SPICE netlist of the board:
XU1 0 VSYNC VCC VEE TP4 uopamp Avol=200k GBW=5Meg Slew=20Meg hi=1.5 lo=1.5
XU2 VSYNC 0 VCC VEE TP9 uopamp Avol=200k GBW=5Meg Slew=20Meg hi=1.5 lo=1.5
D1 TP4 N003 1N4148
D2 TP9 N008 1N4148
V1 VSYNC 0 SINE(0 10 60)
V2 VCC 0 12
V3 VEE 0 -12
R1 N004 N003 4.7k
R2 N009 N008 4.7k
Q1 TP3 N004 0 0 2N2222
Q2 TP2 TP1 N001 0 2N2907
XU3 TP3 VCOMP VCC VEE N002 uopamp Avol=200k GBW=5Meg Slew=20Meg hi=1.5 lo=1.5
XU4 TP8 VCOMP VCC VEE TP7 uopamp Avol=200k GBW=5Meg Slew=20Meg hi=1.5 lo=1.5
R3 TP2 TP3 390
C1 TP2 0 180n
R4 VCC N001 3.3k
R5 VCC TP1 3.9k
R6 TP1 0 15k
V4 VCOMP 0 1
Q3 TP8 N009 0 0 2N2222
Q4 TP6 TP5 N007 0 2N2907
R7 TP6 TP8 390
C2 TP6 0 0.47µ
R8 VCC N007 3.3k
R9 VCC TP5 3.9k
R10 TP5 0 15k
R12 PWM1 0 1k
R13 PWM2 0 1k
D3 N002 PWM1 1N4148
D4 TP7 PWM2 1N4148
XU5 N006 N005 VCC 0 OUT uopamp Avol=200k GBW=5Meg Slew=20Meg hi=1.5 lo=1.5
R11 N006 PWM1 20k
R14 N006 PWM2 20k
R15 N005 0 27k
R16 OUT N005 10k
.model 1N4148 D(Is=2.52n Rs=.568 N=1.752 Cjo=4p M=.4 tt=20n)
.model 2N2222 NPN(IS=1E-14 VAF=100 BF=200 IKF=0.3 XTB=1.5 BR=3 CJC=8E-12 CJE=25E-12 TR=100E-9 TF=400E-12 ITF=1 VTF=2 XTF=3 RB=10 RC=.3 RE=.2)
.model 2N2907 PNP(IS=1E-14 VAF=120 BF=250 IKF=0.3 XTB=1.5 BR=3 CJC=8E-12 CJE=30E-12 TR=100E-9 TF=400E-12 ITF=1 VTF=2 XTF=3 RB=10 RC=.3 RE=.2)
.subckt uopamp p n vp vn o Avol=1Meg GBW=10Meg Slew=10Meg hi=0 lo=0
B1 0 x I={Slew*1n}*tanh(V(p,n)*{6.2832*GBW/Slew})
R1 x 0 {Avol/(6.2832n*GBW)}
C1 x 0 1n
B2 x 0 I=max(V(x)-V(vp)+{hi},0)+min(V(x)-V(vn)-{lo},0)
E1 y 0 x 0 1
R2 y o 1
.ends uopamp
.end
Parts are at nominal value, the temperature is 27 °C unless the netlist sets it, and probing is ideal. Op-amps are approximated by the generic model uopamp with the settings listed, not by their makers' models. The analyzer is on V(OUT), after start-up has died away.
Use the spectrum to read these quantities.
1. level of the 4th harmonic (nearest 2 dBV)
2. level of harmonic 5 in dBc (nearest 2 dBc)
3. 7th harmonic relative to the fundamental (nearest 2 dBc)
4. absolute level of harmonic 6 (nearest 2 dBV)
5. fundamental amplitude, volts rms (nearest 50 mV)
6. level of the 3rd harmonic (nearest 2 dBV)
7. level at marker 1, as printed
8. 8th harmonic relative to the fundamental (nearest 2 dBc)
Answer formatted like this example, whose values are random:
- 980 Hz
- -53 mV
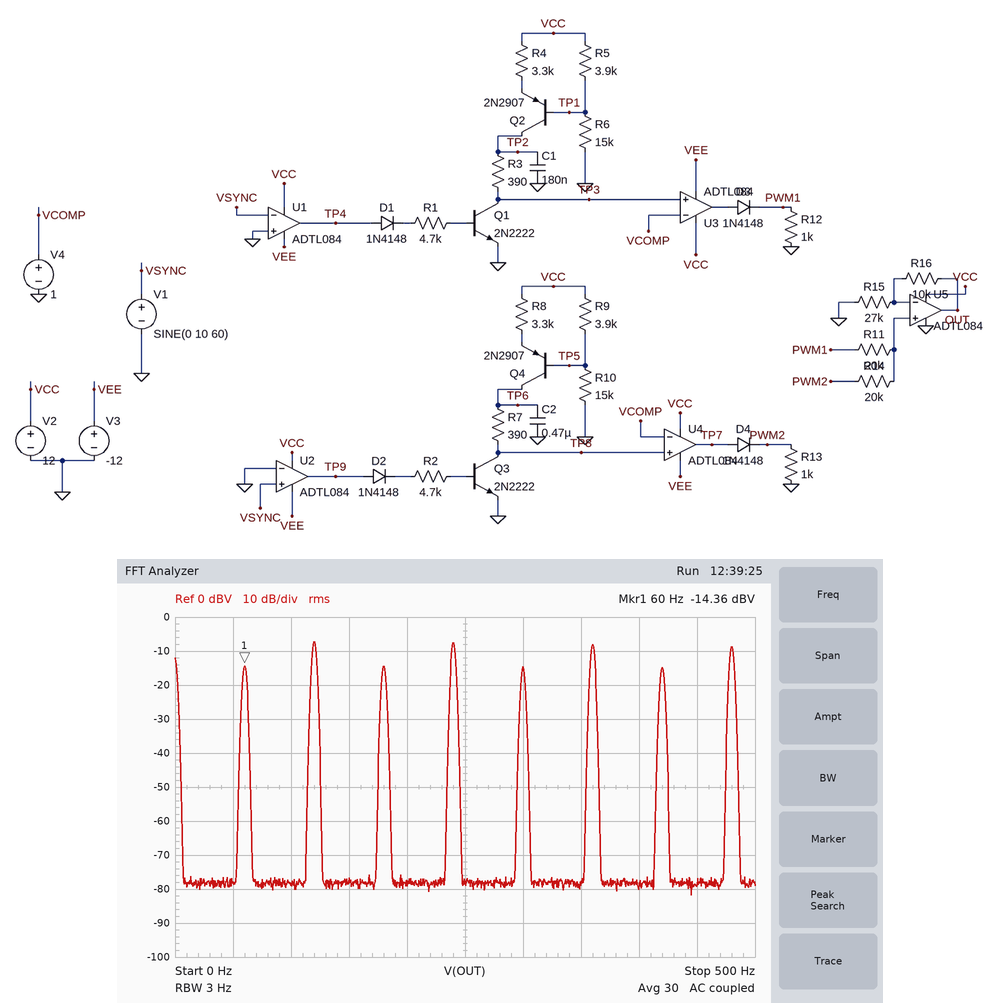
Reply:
- -8 dBV
- 0 dBc
- 0 dBc
- -8 dBV
- 200 mV
- -14 dBV
- -14.36 dBV
- 6 dBc
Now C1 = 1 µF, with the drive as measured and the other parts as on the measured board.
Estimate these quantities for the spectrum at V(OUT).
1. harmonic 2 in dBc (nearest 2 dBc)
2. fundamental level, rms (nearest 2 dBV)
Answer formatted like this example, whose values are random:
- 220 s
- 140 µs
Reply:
- 8 dBc
- -10 dBV
